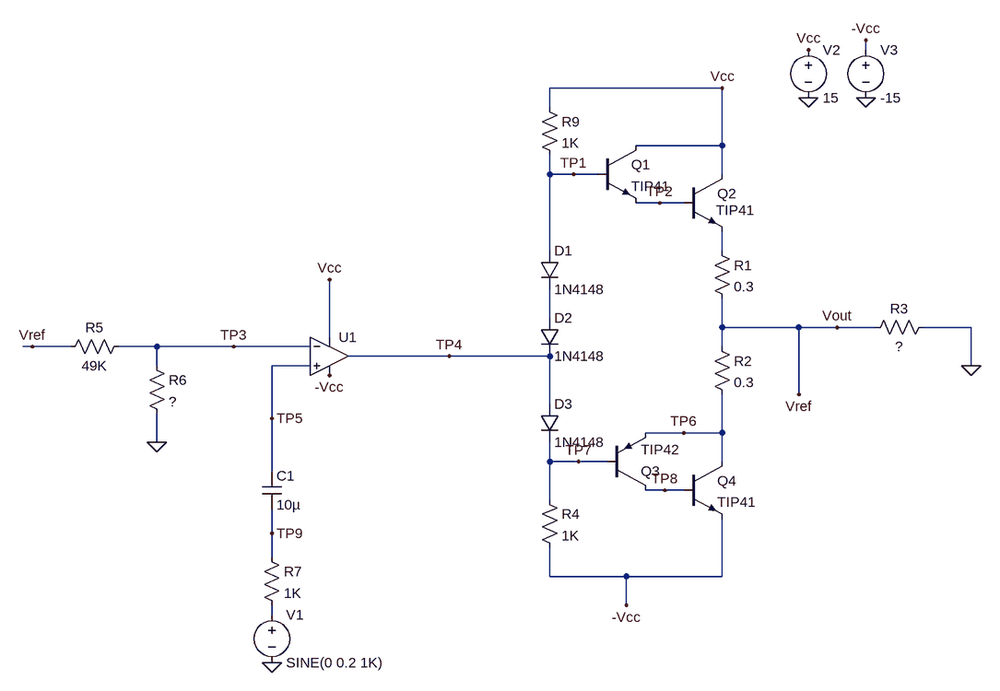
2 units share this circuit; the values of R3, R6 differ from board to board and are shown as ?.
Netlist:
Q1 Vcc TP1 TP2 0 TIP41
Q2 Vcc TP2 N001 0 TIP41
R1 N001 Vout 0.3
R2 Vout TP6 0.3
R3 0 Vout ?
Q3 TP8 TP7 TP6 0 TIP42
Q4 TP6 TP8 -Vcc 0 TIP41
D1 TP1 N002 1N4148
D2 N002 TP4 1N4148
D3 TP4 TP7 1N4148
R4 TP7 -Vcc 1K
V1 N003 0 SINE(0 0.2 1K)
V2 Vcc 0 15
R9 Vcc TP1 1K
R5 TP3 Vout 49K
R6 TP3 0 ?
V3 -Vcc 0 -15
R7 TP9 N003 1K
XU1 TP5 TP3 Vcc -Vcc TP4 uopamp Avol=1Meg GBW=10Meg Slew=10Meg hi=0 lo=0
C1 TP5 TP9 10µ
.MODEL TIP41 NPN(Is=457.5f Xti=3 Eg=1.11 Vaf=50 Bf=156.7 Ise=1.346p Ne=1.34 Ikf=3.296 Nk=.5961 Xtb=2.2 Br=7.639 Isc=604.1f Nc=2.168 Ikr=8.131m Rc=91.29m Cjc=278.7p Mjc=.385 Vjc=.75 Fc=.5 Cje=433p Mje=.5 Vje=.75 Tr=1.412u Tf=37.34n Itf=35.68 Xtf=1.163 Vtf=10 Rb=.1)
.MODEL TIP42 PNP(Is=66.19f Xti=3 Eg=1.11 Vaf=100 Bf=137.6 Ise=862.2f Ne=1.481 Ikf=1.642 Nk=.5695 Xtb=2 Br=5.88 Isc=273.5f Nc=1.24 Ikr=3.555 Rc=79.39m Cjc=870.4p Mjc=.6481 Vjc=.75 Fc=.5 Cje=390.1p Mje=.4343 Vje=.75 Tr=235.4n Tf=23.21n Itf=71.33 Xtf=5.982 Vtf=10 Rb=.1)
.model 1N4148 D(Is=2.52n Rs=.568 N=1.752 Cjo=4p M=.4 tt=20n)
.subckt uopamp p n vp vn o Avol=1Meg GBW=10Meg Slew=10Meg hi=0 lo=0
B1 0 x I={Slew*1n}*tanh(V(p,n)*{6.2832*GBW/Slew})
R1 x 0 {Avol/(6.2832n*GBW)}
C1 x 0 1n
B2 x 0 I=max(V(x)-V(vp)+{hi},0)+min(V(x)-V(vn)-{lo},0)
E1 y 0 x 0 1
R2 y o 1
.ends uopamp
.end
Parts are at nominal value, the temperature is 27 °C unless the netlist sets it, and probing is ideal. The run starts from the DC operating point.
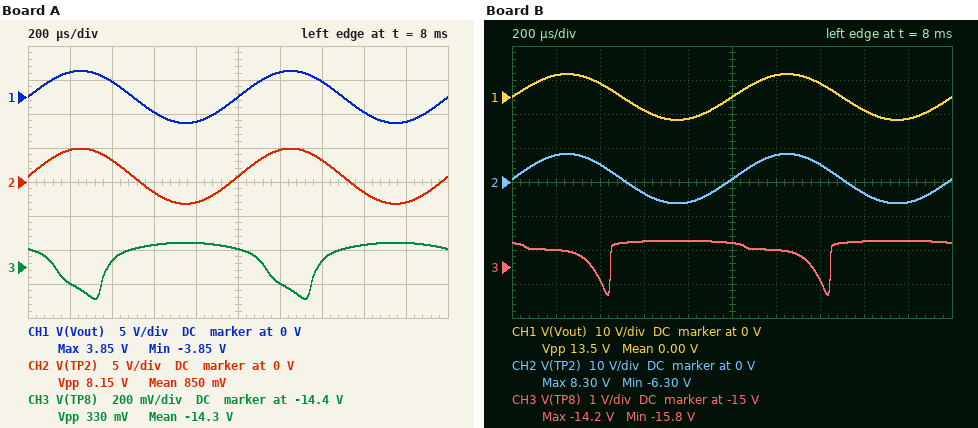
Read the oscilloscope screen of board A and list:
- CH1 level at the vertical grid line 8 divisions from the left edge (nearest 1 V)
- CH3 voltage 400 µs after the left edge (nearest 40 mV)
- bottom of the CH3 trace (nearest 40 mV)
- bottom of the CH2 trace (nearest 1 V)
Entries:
-2 V
-14.36 V
-14.60 V
-3 V
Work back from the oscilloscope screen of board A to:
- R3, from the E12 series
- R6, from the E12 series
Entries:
3.3 Ω
2.7 kΩ
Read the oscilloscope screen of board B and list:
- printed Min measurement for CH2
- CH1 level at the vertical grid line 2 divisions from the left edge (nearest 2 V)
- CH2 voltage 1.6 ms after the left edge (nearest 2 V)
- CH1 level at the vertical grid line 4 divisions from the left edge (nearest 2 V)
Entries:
-6.30 V
4 V
-4 V
-6 V
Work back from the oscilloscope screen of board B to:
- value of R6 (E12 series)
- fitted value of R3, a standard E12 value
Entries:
1.5 kΩ
2.7 Ω
